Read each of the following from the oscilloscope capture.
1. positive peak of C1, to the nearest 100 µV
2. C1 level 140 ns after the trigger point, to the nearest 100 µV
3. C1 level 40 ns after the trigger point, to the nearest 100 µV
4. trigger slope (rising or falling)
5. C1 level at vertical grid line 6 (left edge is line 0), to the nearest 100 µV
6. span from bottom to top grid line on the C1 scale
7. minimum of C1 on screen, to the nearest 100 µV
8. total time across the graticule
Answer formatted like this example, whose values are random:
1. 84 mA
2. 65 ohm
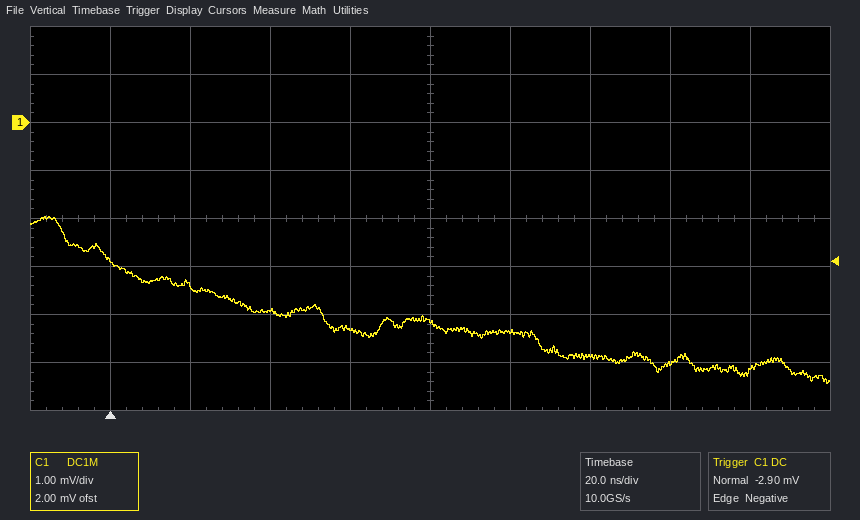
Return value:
1. -2.0 mV
2. -5.0 mV
3. -3.9 mV
4. falling
5. -4.4 mV
6. 8 mV
7. -5.4 mV
8. 200 ns
